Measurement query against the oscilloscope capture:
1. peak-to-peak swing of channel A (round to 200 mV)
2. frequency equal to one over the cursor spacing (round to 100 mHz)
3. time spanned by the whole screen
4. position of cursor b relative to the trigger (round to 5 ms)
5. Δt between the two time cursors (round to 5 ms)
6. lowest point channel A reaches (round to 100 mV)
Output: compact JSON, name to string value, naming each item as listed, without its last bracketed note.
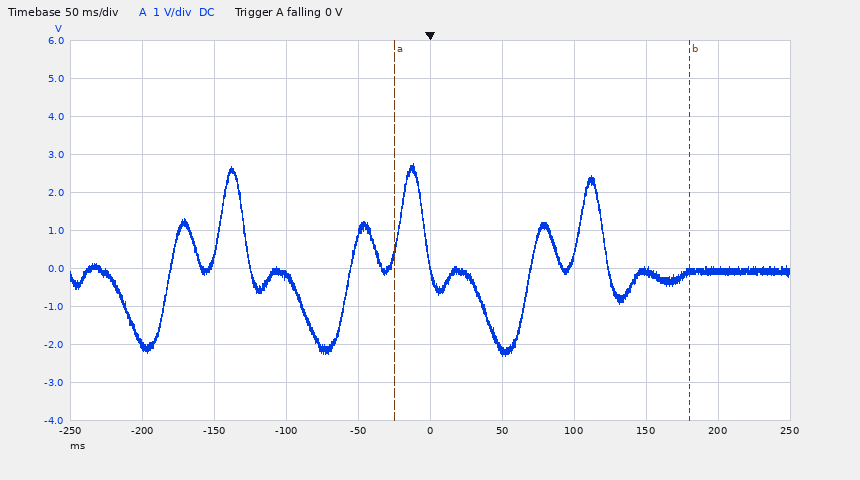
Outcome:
{"peak-to-peak swing of channel A": "5.0 V", "frequency equal to one over the cursor spacing": "4.9 Hz", "time spanned by the whole screen": "500 ms", "position of cursor b relative to the trigger": "+180 ms", "Δt between the two time cursors": "205 ms", "lowest point channel A reaches": "-2.3 V"}
